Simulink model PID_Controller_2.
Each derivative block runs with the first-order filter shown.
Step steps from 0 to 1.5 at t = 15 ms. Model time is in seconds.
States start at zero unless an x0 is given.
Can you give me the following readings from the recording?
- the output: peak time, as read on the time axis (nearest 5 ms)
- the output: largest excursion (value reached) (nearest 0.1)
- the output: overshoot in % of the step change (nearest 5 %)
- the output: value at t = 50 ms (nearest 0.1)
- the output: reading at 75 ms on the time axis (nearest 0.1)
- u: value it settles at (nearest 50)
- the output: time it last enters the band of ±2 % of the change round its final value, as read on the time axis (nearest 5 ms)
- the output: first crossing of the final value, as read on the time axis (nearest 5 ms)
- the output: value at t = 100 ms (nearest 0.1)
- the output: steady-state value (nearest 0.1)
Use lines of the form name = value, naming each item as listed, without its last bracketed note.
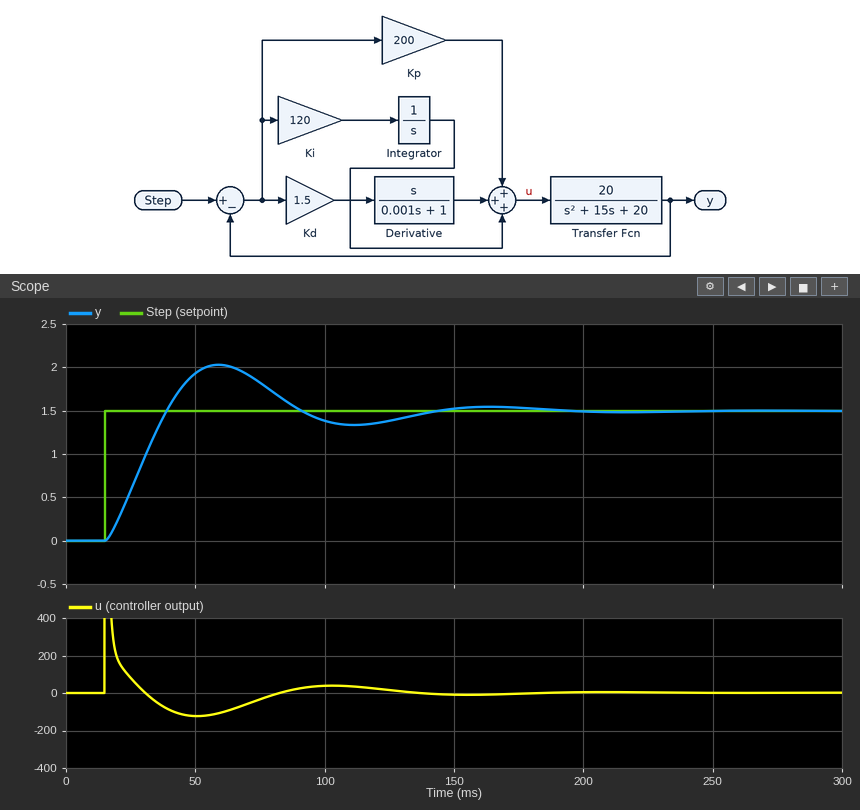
the output: peak time, as read on the time axis = 60 ms
the output: largest excursion (value reached) = 2.0
the output: overshoot in % of the step change = 35 %
the output: value at t = 50 ms = 1.9
the output: reading at 75 ms on the time axis = 1.8
u: value it settles at = 0
the output: time it last enters the band of ±2 % of the change round its final value, as read on the time axis = 180 ms
the output: first crossing of the final value, as read on the time axis = 40 ms
the output: value at t = 100 ms = 1.4
the output: steady-state value = 1.5
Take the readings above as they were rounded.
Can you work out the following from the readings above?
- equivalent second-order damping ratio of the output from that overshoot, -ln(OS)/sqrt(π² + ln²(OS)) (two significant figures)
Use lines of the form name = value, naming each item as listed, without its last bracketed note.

equivalent second-order damping ratio of the output from that overshoot, -ln(OS)/sqrt(π² + ln²(OS)) = 0.32
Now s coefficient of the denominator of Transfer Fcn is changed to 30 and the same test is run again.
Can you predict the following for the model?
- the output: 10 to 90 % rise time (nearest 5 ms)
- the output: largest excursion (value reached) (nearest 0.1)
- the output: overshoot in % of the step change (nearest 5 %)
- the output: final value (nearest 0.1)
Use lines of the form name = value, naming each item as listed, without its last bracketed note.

the output: 10 to 90 % rise time = 20 ms
the output: largest excursion (value reached) = 1.8
the output: overshoot in % of the step change = 20 %
the output: final value = 1.5
